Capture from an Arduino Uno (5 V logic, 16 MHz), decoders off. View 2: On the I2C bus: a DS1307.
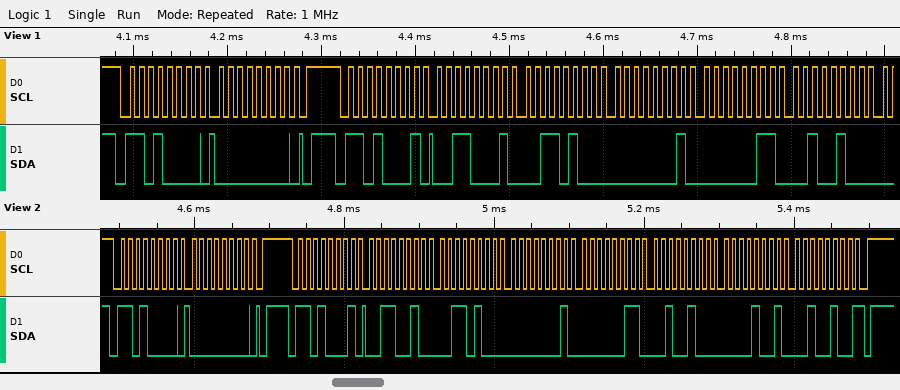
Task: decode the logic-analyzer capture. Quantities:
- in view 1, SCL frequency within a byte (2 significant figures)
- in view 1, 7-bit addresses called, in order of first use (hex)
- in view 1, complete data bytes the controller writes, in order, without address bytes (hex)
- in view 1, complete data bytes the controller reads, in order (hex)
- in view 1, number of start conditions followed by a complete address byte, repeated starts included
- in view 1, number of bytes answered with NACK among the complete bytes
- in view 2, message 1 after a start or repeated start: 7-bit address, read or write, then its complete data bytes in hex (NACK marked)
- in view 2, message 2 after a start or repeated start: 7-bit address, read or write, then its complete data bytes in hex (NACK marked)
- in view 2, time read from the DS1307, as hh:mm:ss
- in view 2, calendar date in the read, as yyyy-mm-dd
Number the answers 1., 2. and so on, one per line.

1. 100 kHz
2. 0x68
3. 00
4. 31 34 01 03 24
5. 2
6. 0
7. 0x68 write: 00
8. 0x68 read: 32 34 01 03 24 09 24 NACK
9. 01:34:32
10. 2024-09-24
